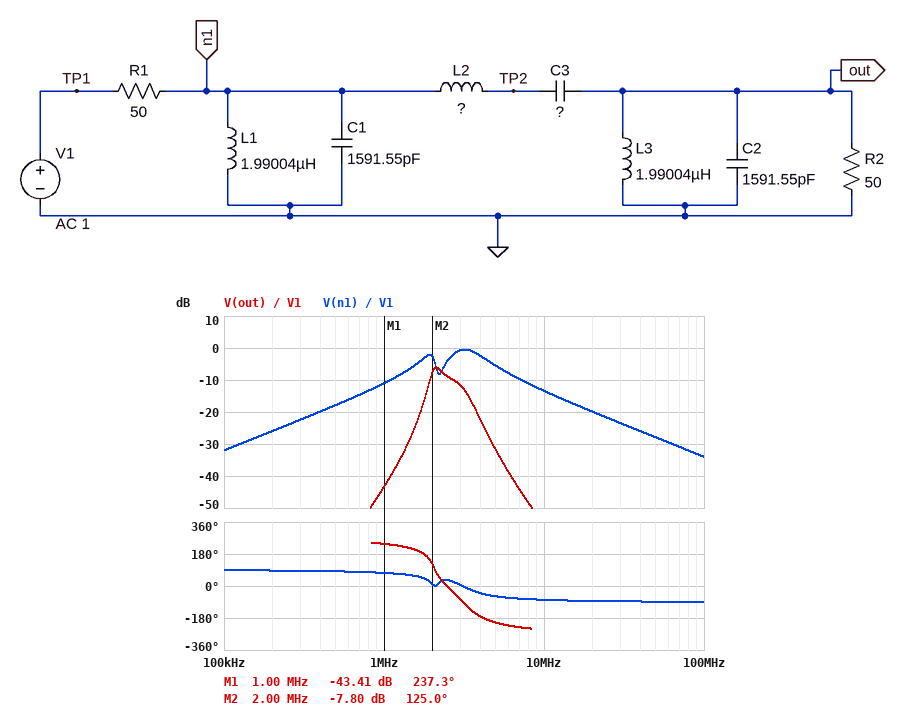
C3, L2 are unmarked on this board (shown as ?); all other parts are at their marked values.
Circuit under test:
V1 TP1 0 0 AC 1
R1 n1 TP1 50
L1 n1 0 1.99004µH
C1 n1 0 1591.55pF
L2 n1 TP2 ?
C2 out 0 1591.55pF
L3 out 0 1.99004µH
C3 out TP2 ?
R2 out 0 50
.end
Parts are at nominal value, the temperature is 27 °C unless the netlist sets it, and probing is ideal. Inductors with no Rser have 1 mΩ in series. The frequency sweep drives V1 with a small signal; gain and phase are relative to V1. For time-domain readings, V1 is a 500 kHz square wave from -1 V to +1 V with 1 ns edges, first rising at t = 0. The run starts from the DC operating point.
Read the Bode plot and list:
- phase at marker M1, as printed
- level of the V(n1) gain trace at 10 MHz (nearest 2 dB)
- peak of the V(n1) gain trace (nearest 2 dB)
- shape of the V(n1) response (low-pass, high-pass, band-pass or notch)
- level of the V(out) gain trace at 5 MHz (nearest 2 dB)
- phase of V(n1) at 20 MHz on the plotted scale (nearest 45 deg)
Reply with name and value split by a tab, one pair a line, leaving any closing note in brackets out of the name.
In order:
phase at marker M1, as printed	237.3 deg
level of the V(n1) gain trace at 10 MHz	-14 dB
peak of the V(n1) gain trace	0 dB
shape of the V(n1) response	band-pass
level of the V(out) gain trace at 5 MHz	-32 dB
phase of V(n1) at 20 MHz on the plotted scale	-90 deg
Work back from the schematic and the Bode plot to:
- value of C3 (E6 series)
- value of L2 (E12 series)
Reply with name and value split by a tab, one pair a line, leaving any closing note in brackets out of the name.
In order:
value of C3	220 pF
value of L2	22 µH
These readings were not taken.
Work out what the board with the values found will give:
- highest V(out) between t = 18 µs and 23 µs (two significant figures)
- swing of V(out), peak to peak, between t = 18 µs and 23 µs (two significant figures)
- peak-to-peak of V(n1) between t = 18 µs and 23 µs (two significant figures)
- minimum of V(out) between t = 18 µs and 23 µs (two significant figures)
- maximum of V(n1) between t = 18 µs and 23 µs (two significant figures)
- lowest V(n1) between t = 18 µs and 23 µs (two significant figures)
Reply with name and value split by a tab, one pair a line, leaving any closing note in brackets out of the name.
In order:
highest V(out) between t = 18 µs and 23 µs	120 mV
swing of V(out), peak to peak, between t = 18 µs and 23 µs	250 mV
peak-to-peak of V(n1) between t = 18 µs and 23 µs	1.7 V
minimum of V(out) between t = 18 µs and 23 µs	-120 mV
maximum of V(n1) between t = 18 µs and 23 µs	870 mV
lowest V(n1) between t = 18 µs and 23 µs	-870 mV
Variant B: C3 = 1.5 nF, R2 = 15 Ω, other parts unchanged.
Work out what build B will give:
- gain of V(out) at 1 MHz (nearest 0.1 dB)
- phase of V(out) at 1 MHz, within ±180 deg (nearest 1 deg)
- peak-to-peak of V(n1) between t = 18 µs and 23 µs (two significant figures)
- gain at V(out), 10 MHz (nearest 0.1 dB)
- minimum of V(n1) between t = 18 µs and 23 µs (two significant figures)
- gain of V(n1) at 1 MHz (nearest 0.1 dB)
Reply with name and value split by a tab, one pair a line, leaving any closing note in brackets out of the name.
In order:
gain of V(out) at 1 MHz	-25.6 dB
phase of V(out) at 1 MHz, within ±180 deg	42 deg
peak-to-peak of V(n1) between t = 18 µs and 23 µs	1.8 V
gain at V(out), 10 MHz	-57.2 dB
minimum of V(n1) between t = 18 µs and 23 µs	-880 mV
gain of V(n1) at 1 MHz	-13.8 dB
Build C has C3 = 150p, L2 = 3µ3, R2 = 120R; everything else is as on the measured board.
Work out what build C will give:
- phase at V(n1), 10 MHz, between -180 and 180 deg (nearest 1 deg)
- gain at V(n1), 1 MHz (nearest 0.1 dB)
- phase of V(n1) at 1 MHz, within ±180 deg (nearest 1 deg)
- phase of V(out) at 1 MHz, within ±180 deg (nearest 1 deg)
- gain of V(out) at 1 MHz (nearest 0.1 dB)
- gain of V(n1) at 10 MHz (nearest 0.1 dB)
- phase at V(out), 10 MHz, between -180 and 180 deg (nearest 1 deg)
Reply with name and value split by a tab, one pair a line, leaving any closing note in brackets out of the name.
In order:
phase at V(n1), 10 MHz, between -180 and 180 deg	-76 deg
gain at V(n1), 1 MHz	-11.1 dB
phase of V(n1) at 1 MHz, within ±180 deg	74 deg
phase of V(out) at 1 MHz, within ±180 deg	-113 deg
gain of V(out) at 1 MHz	-48.3 dB
gain of V(n1) at 10 MHz	-12.4 dB
phase at V(out), 10 MHz, between -180 and 180 deg	110 deg
